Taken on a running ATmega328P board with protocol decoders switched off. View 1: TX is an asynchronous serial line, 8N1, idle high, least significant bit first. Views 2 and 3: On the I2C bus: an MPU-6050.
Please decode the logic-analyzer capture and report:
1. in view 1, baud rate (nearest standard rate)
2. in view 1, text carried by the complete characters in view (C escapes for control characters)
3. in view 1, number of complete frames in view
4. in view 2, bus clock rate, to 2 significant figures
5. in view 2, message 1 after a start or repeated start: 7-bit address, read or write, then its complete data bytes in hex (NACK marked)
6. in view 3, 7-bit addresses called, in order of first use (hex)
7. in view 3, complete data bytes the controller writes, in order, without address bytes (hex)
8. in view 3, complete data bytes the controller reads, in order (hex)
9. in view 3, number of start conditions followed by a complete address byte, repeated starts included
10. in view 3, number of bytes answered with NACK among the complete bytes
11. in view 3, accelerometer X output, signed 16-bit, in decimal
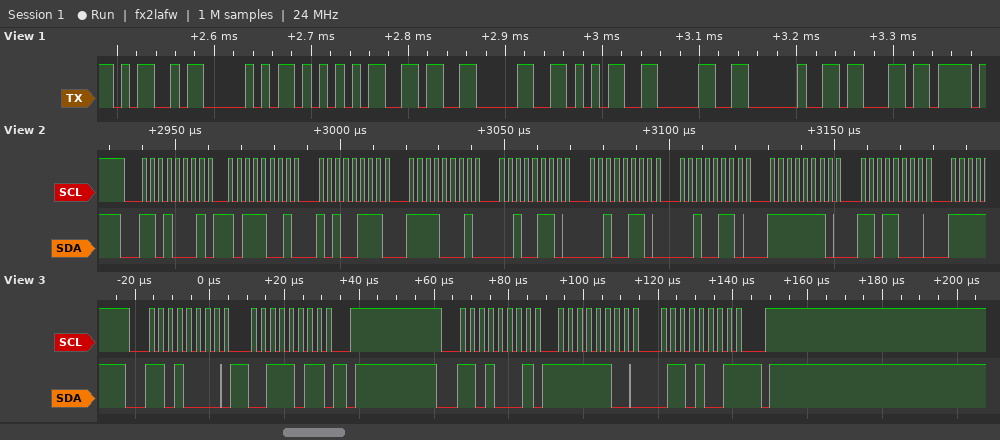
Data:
115200 baud
"MPU6050 c"
9
400 kHz
0x68 read: B9 A7 F1 26 26 26 FE D8
0x68
3B
FC 69
2
1
-919
